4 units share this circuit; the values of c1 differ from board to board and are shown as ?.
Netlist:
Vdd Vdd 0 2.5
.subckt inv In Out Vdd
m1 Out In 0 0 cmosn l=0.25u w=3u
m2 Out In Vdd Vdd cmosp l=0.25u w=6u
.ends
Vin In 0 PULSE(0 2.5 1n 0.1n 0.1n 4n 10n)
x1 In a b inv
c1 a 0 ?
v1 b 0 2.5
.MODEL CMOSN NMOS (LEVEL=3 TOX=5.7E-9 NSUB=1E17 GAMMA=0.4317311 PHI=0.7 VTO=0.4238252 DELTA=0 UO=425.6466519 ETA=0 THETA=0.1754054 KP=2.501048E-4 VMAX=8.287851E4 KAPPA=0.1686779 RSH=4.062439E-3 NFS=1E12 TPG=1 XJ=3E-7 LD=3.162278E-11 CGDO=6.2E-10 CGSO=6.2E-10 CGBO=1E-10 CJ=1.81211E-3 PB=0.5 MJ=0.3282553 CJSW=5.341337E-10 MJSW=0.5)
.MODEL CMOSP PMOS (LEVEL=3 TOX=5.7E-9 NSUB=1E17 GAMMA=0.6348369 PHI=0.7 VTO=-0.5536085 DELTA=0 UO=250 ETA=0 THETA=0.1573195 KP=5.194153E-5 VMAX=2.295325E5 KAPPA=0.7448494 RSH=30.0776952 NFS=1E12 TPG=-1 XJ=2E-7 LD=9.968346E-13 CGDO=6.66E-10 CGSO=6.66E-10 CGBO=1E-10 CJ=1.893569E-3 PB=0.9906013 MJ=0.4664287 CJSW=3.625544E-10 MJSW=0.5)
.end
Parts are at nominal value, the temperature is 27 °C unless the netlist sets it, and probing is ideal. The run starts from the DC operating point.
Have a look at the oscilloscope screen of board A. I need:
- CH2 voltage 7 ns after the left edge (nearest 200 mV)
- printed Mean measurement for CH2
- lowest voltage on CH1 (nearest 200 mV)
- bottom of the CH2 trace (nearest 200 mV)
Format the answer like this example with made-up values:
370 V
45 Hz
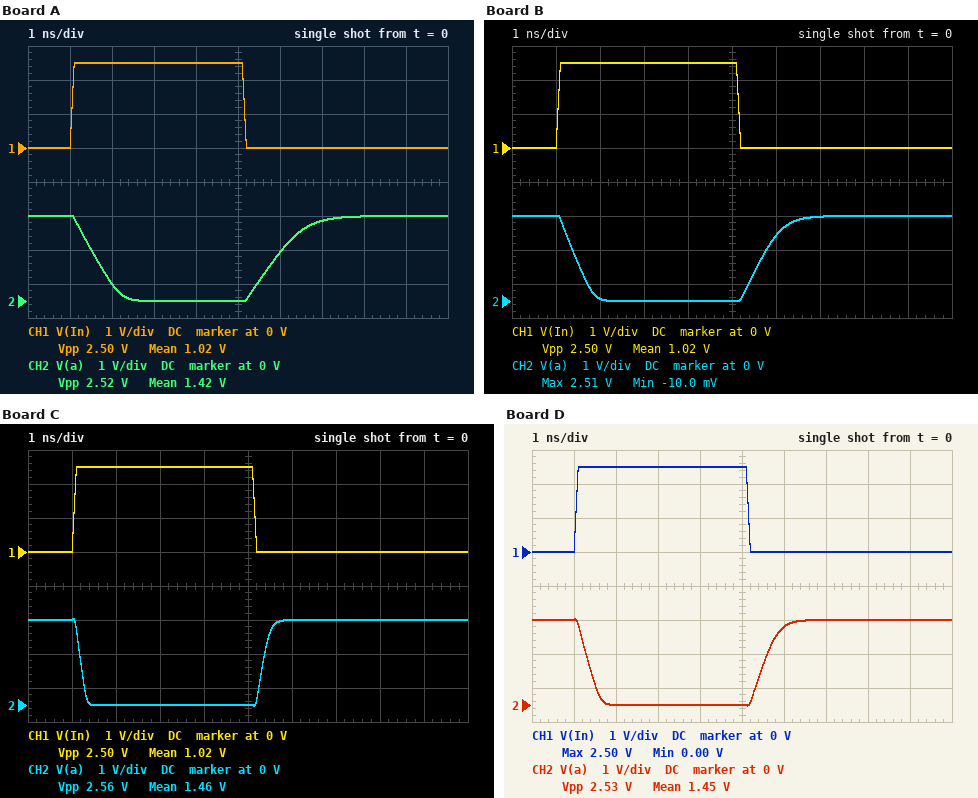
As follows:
2.4 V
1.42 V
0 V
0 V
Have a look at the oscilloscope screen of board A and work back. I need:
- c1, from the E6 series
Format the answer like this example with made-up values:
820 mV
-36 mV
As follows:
680 fF
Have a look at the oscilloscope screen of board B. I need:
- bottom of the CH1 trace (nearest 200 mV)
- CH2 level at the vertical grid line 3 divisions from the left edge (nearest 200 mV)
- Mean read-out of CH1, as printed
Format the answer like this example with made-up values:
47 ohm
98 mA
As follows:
0 V
0 V
1.02 V
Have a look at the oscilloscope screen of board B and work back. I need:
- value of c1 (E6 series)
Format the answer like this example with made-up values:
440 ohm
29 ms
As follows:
470 fF
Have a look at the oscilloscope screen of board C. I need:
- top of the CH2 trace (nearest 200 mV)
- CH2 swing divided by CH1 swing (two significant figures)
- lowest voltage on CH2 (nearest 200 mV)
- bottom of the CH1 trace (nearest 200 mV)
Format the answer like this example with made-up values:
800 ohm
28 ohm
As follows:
2.6 V
1.0
0 V
0 V
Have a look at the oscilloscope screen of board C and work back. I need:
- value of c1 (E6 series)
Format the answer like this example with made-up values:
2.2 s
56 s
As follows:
150 fF
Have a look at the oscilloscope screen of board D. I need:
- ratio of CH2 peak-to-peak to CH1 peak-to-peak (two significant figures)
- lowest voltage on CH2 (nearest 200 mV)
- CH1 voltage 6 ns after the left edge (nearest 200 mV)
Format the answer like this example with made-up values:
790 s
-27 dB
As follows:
1.0
0 V
0 V
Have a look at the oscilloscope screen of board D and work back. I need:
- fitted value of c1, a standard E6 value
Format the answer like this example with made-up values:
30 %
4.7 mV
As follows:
330 fF
